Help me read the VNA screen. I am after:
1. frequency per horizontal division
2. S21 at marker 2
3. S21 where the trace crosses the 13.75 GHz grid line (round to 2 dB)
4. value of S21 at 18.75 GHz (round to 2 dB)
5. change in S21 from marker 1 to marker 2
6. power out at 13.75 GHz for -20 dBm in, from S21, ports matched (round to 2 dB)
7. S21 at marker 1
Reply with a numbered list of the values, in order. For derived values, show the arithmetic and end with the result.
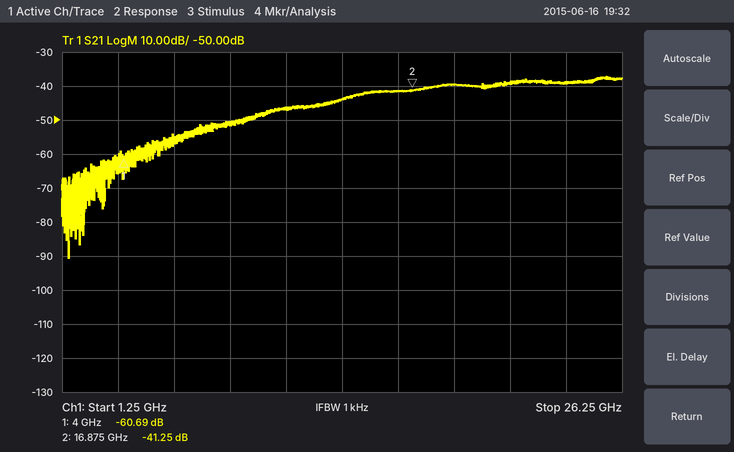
1. 2.5 GHz
2. -41.25 dB
3. -44 dB
4. -40 dB
5. -41.25 − (-60.69) = 19.44 dB
6. -20 dBm + (-44 dB) = -64 dBm
7. -60.69 dB
